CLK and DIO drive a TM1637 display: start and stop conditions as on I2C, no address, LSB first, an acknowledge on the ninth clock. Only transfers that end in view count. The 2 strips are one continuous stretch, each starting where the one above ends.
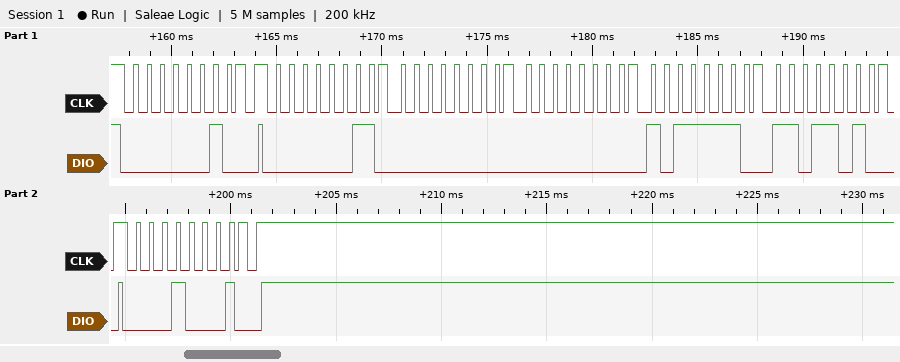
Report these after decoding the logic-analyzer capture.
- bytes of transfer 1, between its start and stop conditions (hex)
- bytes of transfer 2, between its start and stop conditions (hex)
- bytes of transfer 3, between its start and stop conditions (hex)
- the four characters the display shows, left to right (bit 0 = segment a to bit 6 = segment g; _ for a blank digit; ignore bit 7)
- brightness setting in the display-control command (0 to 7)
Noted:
40
C0 00 00 7D 5B
88
__62
0
